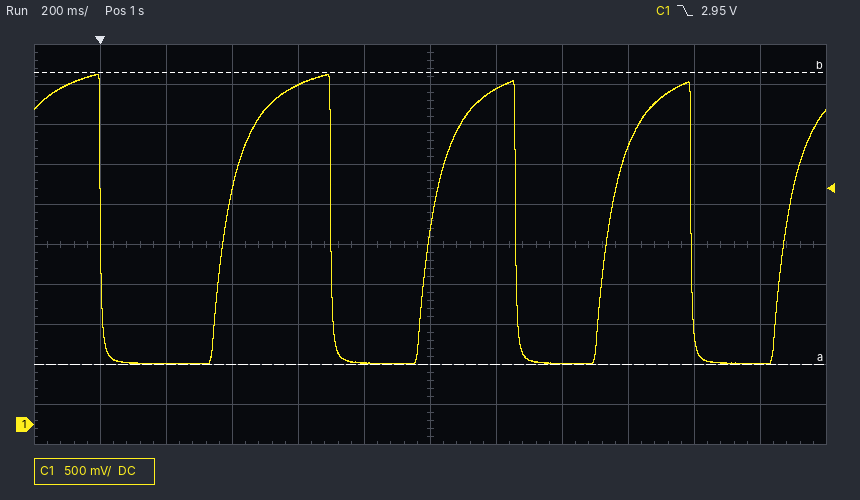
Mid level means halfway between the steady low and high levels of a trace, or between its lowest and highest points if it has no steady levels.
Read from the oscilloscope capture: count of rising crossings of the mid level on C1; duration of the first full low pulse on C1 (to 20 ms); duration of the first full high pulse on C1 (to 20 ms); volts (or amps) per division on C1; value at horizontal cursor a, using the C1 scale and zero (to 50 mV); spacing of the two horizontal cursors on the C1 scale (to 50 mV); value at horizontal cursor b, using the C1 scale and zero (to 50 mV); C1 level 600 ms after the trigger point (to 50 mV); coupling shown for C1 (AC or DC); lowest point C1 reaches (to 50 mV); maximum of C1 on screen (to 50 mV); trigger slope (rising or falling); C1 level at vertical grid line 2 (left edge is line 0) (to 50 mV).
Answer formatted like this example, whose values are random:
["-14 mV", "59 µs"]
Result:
["4", "380 ms", "320 ms", "500 mV", "750 mV", "3.65 V", "4.40 V", "4.25 V", "DC", "750 mV", "4.40 V", "falling", "750 mV"]
